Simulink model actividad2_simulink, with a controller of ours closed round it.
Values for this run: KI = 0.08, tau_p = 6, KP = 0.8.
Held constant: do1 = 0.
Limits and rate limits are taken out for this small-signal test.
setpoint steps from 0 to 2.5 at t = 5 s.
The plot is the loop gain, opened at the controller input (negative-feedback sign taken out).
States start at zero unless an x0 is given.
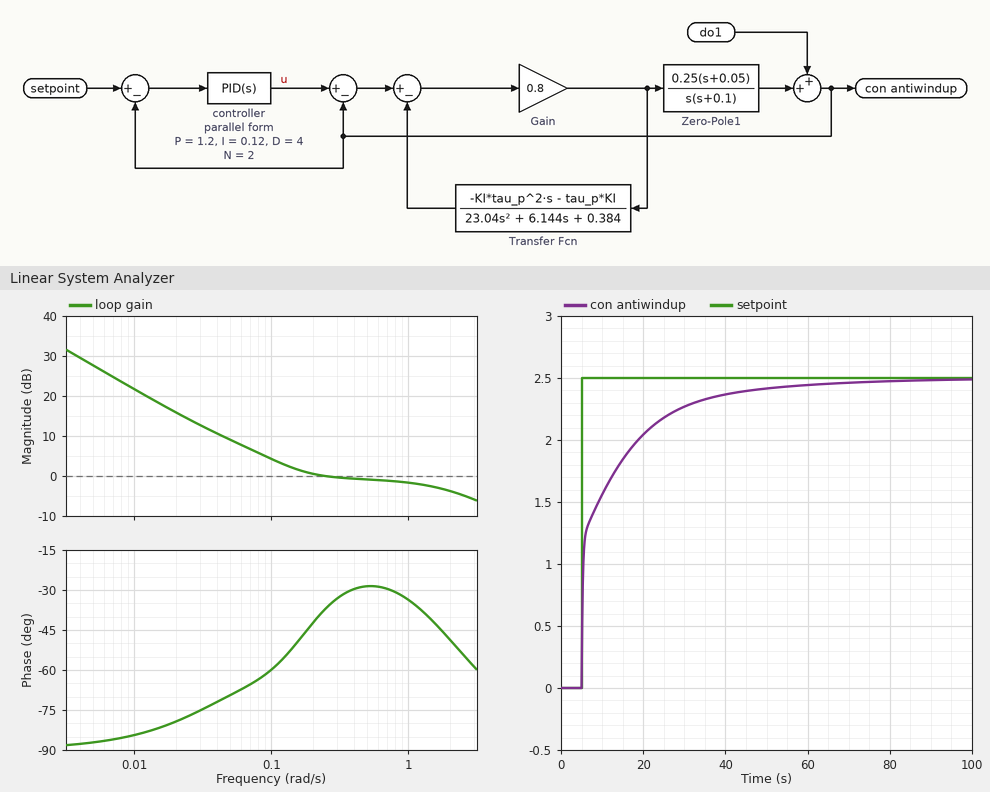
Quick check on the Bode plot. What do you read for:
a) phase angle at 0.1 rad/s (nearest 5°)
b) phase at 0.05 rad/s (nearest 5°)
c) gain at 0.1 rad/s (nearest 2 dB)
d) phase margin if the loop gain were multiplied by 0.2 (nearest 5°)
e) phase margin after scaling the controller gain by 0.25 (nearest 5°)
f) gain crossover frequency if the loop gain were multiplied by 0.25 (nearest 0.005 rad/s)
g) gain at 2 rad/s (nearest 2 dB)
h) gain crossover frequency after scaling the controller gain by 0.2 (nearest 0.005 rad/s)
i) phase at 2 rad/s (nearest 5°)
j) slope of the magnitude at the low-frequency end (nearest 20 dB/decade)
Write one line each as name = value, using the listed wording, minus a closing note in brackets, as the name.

phase angle at 0.1 rad/s = -60°
phase at 0.05 rad/s = -70°
gain at 0.1 rad/s = 4 dB
phase margin if the loop gain were multiplied by 0.2 = 105°
phase margin after scaling the controller gain by 0.25 = 105°
gain crossover frequency if the loop gain were multiplied by 0.25 = 0.035 rad/s
gain at 2 rad/s = -4 dB
gain crossover frequency after scaling the controller gain by 0.2 = 0.025 rad/s
phase at 2 rad/s = -50°
slope of the magnitude at the low-frequency end = -20 dB/decade
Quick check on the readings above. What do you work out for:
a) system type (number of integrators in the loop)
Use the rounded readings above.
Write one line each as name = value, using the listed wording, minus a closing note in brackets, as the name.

system type = 1
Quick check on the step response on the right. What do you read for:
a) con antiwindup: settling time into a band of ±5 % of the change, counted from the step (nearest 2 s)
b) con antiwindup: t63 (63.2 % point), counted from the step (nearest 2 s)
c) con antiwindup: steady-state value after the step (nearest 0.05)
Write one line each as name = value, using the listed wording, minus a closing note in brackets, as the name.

con antiwindup: settling time into a band of ±5 % of the change, counted from the step = 36 s
con antiwindup: t63 (63.2 % point), counted from the step = 6 s
con antiwindup: steady-state value after the step = 2.50
